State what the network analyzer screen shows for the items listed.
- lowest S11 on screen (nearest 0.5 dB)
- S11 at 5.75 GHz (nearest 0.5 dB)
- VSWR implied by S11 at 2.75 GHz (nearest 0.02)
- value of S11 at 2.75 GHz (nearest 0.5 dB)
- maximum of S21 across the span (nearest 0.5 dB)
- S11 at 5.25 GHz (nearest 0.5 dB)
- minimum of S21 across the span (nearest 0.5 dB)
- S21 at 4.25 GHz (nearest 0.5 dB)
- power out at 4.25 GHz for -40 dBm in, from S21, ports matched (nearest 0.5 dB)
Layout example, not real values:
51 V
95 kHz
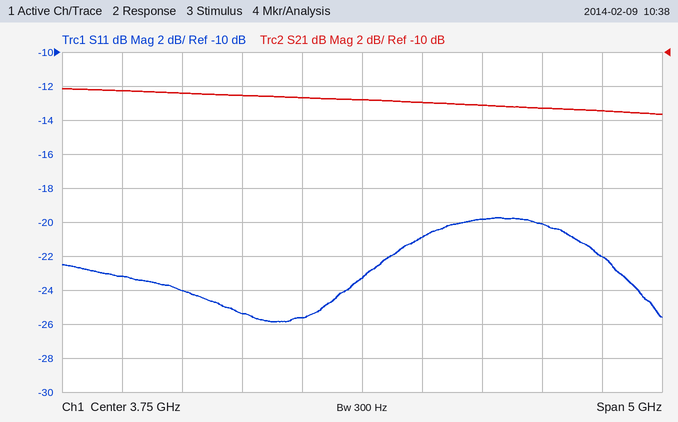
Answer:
-26.0 dB
-22.0 dB
1.12
-25.5 dB
-12.0 dB
-20.0 dB
-13.5 dB
-13.0 dB
-53.0 dBm
